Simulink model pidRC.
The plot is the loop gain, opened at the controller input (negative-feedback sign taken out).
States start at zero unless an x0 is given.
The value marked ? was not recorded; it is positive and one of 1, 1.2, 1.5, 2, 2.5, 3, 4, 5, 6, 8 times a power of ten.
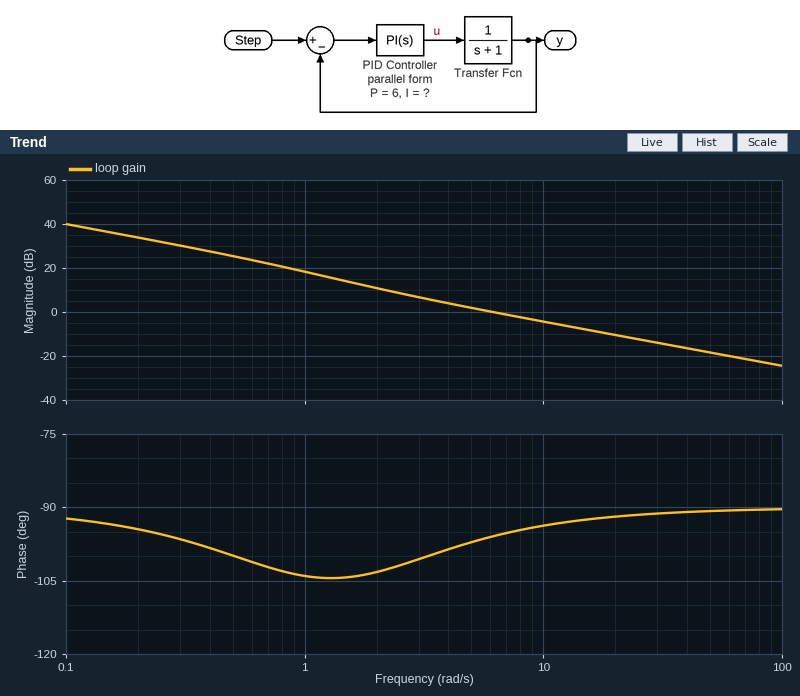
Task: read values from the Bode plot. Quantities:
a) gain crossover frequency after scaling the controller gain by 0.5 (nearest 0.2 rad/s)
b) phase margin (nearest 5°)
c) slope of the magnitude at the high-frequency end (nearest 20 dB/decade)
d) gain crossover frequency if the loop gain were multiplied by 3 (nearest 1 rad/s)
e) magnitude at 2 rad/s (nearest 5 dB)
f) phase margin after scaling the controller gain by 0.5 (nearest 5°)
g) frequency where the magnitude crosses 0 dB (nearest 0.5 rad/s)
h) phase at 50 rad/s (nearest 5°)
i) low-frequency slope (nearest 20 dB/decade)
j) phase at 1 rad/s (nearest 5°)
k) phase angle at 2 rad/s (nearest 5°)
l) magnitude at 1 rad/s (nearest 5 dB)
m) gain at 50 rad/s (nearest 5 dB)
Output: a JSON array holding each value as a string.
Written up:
["3.2 rad/s", "85°", "-20 dB/decade", "18 rad/s", "10 dB", "80°", "6.0 rad/s", "-90°", "-20 dB/decade", "-105°", "-105°", "20 dB", "-20 dB"]
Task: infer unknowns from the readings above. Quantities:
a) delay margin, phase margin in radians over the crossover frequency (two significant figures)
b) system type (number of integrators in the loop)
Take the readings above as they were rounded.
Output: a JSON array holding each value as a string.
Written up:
["0.25 s", "1"]
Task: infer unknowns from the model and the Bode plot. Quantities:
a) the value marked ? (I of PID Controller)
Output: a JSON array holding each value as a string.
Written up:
["10"]
